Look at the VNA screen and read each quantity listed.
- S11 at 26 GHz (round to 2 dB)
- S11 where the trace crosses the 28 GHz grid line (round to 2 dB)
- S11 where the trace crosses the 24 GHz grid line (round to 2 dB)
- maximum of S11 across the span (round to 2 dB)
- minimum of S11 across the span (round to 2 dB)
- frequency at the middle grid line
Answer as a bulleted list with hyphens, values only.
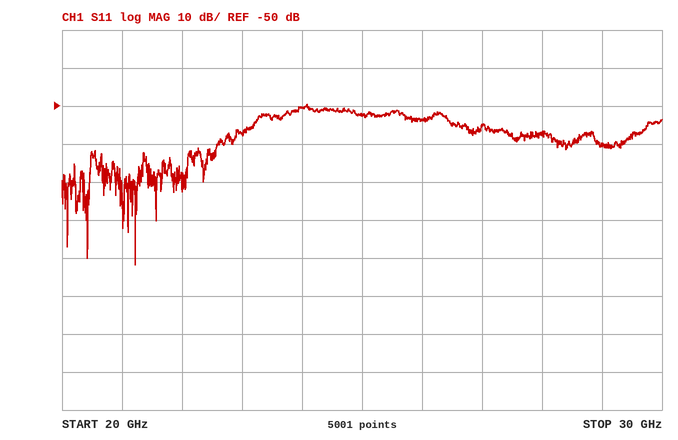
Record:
- -54 dB
- -58 dB
- -50 dB
- -50 dB
- -92 dB
- 25 GHz
